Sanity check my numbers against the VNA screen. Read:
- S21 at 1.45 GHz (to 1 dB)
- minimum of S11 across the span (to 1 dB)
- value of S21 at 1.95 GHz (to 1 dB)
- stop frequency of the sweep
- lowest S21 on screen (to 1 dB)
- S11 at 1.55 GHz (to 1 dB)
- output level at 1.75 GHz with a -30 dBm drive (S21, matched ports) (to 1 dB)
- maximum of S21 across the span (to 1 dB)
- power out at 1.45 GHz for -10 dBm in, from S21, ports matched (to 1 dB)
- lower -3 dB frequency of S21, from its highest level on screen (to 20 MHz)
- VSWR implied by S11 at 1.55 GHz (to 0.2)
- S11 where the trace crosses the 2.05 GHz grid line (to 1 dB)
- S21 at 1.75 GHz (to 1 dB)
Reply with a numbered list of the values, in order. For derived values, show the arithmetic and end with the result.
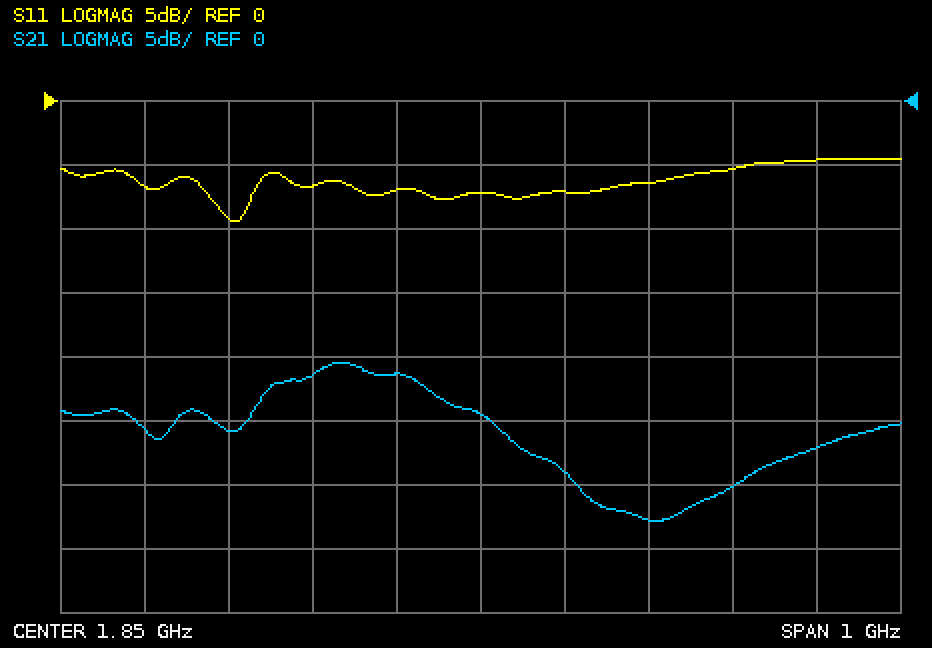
1. -26 dB
2. -9 dB
3. -29 dB
4. 2.35 GHz
5. -33 dB
6. -9 dB
7. -30 dBm + (-21 dB) = -51 dBm
8. -20 dB
9. -10 dBm + (-26 dB) = -36 dBm
10. 1.58 GHz
11. |Γ| = 10^(-9/20) = 0.3548; VSWR = (1 + 0.3548)/(1 − 0.3548) ≈ 2.10, so 2.0 to the nearest 0.2
12. -6 dB
13. -21 dB
